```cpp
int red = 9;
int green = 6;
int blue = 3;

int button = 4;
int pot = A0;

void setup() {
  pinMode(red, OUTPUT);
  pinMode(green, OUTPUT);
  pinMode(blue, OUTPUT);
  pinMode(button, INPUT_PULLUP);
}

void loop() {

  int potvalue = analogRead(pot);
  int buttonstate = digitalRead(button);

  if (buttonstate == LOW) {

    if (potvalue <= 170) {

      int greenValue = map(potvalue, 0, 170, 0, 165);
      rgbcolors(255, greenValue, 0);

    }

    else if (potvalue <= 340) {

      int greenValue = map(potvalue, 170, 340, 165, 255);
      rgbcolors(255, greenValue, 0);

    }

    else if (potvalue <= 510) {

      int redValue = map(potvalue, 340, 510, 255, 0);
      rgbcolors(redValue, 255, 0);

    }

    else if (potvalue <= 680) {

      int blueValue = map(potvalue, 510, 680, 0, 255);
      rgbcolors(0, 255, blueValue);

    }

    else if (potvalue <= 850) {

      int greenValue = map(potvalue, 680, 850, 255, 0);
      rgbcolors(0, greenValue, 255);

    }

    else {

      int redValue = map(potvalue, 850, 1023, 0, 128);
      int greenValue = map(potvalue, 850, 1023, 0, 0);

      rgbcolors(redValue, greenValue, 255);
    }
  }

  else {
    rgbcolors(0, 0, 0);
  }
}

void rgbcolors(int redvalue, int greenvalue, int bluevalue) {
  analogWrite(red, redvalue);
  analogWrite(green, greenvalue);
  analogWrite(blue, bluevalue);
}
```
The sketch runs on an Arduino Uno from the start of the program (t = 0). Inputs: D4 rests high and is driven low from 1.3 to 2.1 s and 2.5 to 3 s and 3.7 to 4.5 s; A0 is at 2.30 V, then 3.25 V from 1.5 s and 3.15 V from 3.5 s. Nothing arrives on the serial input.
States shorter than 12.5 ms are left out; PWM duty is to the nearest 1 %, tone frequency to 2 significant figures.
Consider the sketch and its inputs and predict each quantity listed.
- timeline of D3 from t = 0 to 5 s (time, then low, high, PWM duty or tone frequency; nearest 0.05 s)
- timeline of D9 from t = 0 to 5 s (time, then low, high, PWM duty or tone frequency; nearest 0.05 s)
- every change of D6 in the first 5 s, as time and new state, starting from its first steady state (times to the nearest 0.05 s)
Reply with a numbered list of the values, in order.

1. 0 s low; 1.5 s PWM 91 %; 2.1 s low; 2.5 s PWM 91 %; 3 s low; 3.7 s PWM 79 %; 4.5 s low
2. 0 s low; 1.3 s PWM 23 %; 1.5 s low
3. 0 s low; 1.3 s high; 2.1 s low; 2.5 s high; 3 s low; 3.7 s high; 4.5 s low
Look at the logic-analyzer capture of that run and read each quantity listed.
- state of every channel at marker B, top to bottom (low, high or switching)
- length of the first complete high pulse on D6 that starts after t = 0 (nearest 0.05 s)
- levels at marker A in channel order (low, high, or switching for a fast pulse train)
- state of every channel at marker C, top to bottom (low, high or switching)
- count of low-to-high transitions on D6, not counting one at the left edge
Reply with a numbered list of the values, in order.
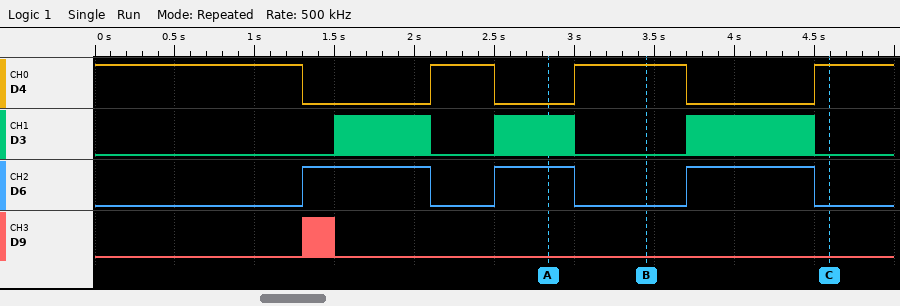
1. D4 high, D3 low, D6 low, D9 low
2. 0.80 s
3. D4 low, D3 switching, D6 high, D9 low
4. D4 high, D3 low, D6 low, D9 low
5. 3
